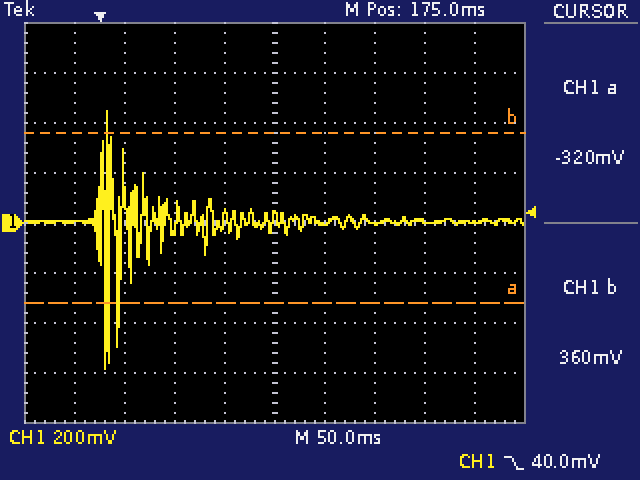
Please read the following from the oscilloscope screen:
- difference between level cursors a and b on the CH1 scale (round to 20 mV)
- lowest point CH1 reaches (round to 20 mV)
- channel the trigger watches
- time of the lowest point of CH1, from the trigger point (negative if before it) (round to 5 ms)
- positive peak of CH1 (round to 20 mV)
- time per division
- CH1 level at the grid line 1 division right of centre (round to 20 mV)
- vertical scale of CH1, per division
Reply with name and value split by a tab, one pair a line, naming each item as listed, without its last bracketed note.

difference between level cursors a and b on the CH1 scale	680 mV
lowest point CH1 reaches	-580 mV
channel the trigger watches	CH1
time of the lowest point of CH1, from the trigger point (negative if before it)	+5 ms
positive peak of CH1	440 mV
time per division	50 ms
CH1 level at the grid line 1 division right of centre	0 mV
vertical scale of CH1, per division	200 mV
